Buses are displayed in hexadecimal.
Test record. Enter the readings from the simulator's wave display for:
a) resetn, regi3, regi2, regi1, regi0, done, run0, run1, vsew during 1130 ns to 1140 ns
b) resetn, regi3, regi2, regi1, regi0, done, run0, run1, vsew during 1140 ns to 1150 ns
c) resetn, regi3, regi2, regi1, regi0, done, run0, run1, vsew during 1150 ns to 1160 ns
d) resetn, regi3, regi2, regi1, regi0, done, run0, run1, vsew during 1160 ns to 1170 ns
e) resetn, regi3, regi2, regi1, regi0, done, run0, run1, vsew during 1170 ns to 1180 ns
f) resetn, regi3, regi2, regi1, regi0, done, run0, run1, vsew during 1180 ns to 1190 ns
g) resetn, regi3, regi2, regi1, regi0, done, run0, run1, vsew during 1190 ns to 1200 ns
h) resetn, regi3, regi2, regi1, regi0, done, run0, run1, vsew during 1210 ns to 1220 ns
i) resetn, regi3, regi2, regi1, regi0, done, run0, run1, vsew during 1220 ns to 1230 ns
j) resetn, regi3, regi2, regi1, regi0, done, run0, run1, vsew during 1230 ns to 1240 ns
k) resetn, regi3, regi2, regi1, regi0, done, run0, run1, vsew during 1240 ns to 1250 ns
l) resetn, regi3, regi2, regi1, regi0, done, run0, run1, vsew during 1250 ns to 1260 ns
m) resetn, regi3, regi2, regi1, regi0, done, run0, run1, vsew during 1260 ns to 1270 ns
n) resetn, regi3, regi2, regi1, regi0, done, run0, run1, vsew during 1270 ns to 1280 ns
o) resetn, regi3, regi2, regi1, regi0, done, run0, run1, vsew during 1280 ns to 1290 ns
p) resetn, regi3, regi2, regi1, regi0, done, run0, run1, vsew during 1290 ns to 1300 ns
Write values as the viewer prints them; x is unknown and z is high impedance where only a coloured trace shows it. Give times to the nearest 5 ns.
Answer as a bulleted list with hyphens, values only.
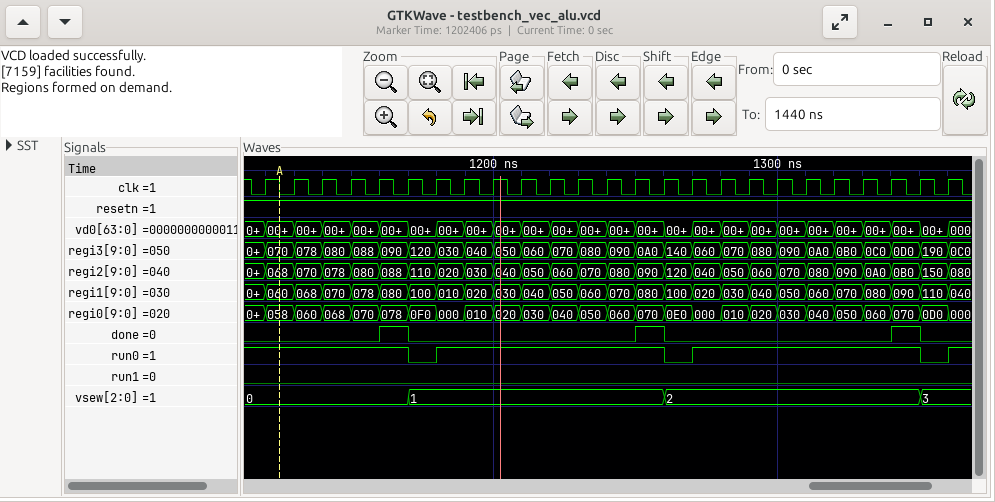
- resetn=1, regi3=078, regi2=070, regi1=068, regi0=060, done=0, run0=1, run1=0, vsew=0
- resetn=1, regi3=080, regi2=078, regi1=070, regi0=068, done=0, run0=1, run1=0, vsew=0
- resetn=1, regi3=088, regi2=080, regi1=078, regi0=070, done=0, run0=1, run1=0, vsew=0
- resetn=1, regi3=090, regi2=088, regi1=080, regi0=078, done=1, run0=1, run1=0, vsew=0
- resetn=1, regi3=120, regi2=110, regi1=100, regi0=0F0, done=0, run0=0, run1=0, vsew=1
- resetn=1, regi3=030, regi2=020, regi1=010, regi0=000, done=0, run0=1, run1=0, vsew=1
- resetn=1, regi3=040, regi2=030, regi1=020, regi0=010, done=0, run0=1, run1=0, vsew=1
- resetn=1, regi3=060, regi2=050, regi1=040, regi0=030, done=0, run0=1, run1=0, vsew=1
- resetn=1, regi3=070, regi2=060, regi1=050, regi0=040, done=0, run0=1, run1=0, vsew=1
- resetn=1, regi3=080, regi2=070, regi1=060, regi0=050, done=0, run0=1, run1=0, vsew=1
- resetn=1, regi3=090, regi2=080, regi1=070, regi0=060, done=0, run0=1, run1=0, vsew=1
- resetn=1, regi3=0A0, regi2=090, regi1=080, regi0=070, done=1, run0=1, run1=0, vsew=1
- resetn=1, regi3=140, regi2=120, regi1=100, regi0=0E0, done=0, run0=0, run1=0, vsew=2
- resetn=1, regi3=060, regi2=040, regi1=020, regi0=000, done=0, run0=1, run1=0, vsew=2
- resetn=1, regi3=070, regi2=050, regi1=030, regi0=010, done=0, run0=1, run1=0, vsew=2
- resetn=1, regi3=080, regi2=060, regi1=040, regi0=020, done=0, run0=1, run1=0, vsew=2
